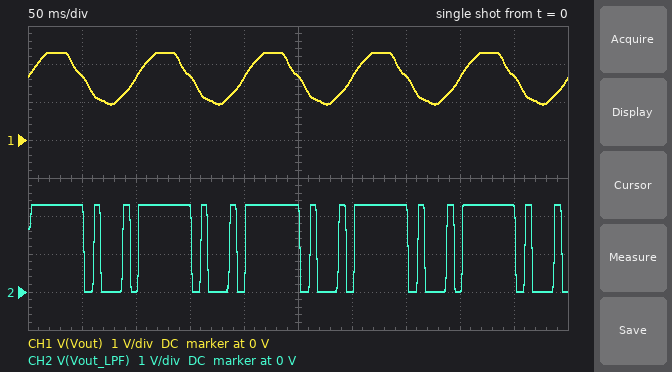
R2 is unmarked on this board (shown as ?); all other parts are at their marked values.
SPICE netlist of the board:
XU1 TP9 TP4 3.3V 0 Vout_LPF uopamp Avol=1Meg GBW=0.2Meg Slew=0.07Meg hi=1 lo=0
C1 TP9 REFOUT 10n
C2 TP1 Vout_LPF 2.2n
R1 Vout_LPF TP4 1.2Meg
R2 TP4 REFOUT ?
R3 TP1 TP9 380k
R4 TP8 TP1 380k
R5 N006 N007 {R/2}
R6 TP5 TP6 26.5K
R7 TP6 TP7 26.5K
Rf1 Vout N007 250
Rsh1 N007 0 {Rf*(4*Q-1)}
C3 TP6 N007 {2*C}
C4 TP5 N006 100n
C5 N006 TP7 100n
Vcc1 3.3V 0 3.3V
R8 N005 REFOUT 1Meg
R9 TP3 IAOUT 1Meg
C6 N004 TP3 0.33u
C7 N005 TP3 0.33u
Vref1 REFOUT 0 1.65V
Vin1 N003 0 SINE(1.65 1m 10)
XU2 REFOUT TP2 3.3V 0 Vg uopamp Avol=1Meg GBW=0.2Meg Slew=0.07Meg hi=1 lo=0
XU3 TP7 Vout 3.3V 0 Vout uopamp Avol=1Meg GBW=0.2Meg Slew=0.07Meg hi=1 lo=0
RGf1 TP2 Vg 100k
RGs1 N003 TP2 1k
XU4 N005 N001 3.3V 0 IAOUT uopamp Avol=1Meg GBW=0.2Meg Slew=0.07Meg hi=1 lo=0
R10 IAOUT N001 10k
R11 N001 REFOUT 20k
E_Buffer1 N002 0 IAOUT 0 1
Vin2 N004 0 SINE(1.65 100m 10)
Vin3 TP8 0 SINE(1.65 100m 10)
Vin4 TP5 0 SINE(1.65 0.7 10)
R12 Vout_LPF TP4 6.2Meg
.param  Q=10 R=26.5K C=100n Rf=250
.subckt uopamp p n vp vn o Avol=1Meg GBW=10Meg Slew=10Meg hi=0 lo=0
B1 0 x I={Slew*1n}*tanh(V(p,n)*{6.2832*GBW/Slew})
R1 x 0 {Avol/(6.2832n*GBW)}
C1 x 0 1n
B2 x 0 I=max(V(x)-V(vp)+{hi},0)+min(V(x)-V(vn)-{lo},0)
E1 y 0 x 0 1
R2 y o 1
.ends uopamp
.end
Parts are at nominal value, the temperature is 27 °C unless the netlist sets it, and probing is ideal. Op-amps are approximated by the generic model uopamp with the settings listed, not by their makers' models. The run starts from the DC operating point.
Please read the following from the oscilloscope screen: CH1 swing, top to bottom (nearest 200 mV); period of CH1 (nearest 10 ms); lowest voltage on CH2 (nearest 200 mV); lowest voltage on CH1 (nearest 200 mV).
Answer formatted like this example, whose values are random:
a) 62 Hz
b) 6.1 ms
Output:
a) 1.4 V
b) 100 ms
c) 0 V
d) 1.0 V
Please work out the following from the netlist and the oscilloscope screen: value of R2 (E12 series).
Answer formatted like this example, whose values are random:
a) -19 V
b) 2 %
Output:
a) 68 kΩ
